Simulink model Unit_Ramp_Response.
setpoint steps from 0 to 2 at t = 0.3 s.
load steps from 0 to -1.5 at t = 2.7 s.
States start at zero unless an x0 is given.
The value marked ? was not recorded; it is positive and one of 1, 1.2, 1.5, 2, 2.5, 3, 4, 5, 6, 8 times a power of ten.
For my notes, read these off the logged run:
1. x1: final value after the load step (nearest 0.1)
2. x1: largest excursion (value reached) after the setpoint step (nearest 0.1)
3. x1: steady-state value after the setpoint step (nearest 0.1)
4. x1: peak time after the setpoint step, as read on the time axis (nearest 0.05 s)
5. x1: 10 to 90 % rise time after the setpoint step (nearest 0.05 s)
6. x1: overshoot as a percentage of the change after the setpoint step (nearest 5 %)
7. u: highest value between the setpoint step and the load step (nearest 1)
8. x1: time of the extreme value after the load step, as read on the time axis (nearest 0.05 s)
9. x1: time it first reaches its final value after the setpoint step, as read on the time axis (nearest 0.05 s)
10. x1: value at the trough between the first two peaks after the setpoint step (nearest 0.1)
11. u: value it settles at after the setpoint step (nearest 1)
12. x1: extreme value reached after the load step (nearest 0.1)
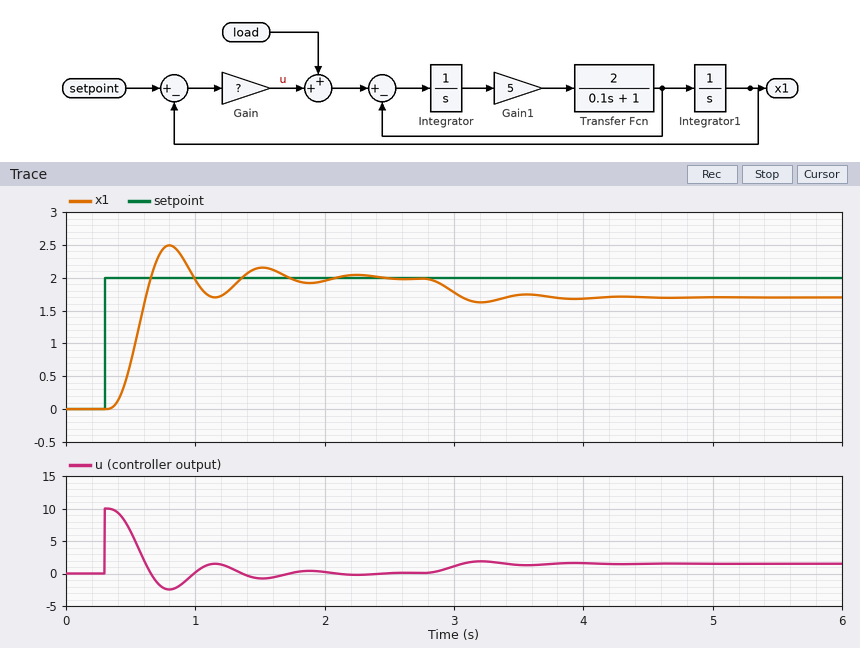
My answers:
1.7
2.5
2.0
0.80 s
0.20 s
25 %
10
3.20 s
0.65 s
1.7
0
1.6
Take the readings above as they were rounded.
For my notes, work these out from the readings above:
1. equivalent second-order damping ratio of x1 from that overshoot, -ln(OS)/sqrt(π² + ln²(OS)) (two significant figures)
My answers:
0.40
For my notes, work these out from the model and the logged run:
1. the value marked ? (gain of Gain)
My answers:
5
